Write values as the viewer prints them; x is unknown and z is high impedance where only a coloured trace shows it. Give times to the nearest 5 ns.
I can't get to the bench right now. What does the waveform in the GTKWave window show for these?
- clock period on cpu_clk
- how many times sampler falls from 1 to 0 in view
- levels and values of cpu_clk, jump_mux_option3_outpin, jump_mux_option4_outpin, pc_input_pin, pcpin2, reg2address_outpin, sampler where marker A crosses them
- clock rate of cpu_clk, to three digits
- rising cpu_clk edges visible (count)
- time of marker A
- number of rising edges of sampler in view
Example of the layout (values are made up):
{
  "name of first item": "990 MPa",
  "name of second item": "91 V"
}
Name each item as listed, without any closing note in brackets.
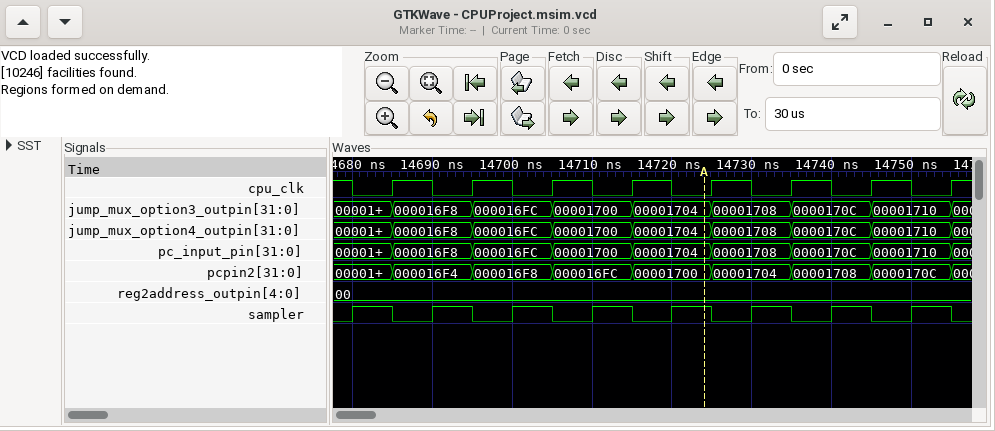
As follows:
{
  "clock period on cpu_clk": "10 ns",
  "how many times sampler falls from 1 to 0 in view": "8",
  "levels and values of cpu_clk, jump_mux_option3_outpin, jump_mux_option4_outpin, pc_input_pin, pcpin2, reg2address_outpin, sampler where marker A crosses them": "cpu_clk=0, jump_mux_option3_outpin=00001704, jump_mux_option4_outpin=00001704, pc_input_pin=00001704, pcpin2=00001700, reg2address_outpin=00, sampler=1",
  "clock rate of cpu_clk, to three digits": "100 MHz",
  "rising cpu_clk edges visible": "8",
  "time of marker A": "14725 ns",
  "number of rising edges of sampler in view": "8"
}
